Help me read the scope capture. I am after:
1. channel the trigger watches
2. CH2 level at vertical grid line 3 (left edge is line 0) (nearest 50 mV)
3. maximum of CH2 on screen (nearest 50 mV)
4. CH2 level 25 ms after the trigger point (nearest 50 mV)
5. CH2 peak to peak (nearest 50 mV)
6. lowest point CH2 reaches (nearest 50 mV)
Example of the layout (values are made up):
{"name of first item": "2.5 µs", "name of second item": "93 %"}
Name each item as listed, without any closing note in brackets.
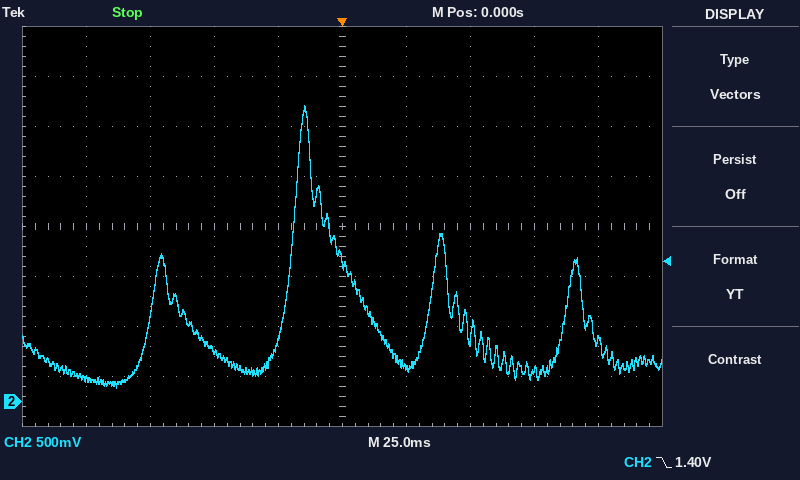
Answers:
{"channel the trigger watches": "CH2", "CH2 level at vertical grid line 3 (left edge is line 0)": "500 mV", "maximum of CH2 on screen": "2.95 V", "CH2 level 25 ms after the trigger point": "350 mV", "CH2 peak to peak": "2.80 V", "lowest point CH2 reaches": "150 mV"}
